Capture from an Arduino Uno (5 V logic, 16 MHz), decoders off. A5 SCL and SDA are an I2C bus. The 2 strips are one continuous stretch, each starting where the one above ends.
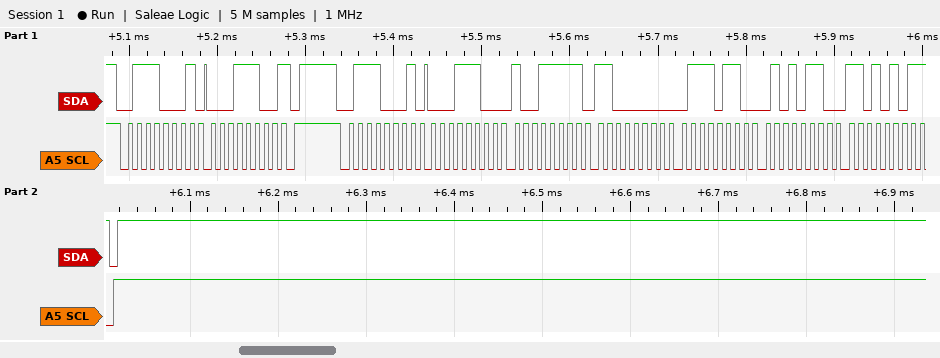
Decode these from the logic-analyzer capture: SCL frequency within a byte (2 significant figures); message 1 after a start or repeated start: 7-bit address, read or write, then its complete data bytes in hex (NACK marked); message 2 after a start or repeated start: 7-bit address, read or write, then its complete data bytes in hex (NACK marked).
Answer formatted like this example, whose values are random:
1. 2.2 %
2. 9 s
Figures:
1. 100 kHz
2. 0x38 read: 1C NACK
3. 0x38 read: 1C 9F C0 76 56 D5 NACK
